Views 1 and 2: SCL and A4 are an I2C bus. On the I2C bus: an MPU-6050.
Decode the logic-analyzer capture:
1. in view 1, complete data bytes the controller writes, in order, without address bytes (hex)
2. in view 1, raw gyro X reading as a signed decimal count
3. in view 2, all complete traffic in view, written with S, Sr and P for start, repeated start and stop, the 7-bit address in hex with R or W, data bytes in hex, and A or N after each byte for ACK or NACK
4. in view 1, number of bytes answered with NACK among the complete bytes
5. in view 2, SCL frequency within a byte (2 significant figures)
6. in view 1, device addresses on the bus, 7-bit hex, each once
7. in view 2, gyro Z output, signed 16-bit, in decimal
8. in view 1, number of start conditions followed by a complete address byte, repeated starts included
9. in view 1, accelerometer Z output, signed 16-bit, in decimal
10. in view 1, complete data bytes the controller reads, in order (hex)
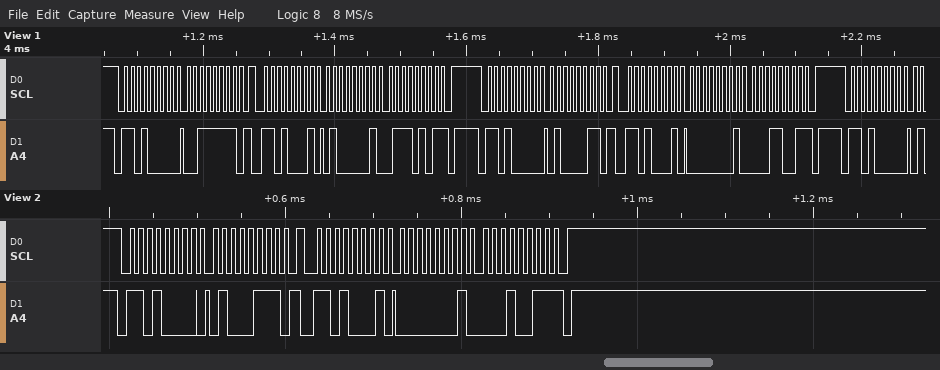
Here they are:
3F 43
281
S 68W A 47 A Sr 68R A 01 A 13 N P
2
100 kHz
0x68
275
5
16757
41 75 01 19
